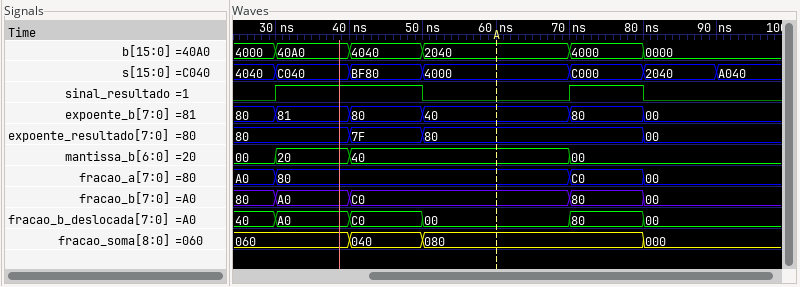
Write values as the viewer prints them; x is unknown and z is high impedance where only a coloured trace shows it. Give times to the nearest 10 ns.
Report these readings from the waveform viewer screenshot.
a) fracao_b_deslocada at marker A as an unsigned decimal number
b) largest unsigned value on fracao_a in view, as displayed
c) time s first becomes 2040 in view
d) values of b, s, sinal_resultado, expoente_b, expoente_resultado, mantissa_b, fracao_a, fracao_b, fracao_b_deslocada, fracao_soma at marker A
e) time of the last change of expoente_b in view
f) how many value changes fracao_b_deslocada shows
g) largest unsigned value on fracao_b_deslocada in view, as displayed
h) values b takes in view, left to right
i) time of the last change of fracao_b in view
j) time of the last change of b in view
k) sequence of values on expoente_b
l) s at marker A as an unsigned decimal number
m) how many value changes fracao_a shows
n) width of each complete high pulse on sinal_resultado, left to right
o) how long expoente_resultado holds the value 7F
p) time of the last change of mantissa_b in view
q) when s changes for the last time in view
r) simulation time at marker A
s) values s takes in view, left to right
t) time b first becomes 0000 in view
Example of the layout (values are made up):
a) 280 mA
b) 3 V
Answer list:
a) 0
b) C0
c) 80 ns
d) b=2040, s=4000, sinal_resultado=0, expoente_b=40, expoente_resultado=80, mantissa_b=40, fracao_a=80, fracao_b=C0, fracao_b_deslocada=00, fracao_soma=080
e) 80 ns
f) 5
g) C0
h) 4000, 40A0, 4040, 2040, 4000, 0000
i) 80 ns
j) 80 ns
k) 80, 81, 80, 40, 80, 00
l) 16384
m) 3
n) 20 ns, 10 ns
o) 10 ns
p) 70 ns
q) 90 ns
r) 60 ns
s) 4040, C040, BF80, 4000, C000, 2040, A040
t) 80 ns
